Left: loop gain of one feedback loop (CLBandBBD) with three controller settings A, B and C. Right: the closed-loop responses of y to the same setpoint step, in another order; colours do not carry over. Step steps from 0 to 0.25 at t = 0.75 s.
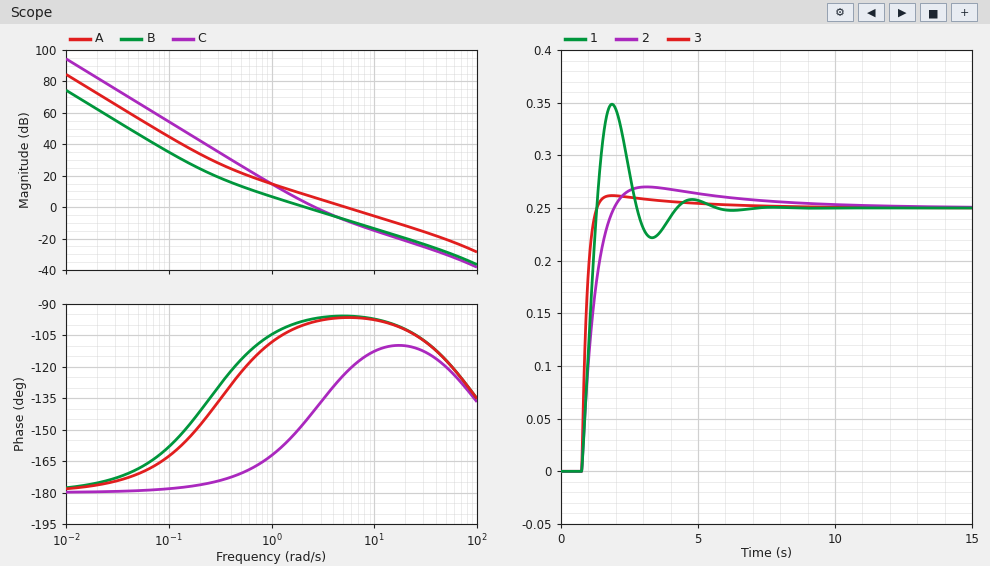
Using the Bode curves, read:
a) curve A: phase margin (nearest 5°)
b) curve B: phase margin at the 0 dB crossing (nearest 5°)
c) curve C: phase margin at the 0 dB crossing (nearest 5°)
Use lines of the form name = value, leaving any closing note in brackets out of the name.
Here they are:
curve A: phase margin = 85°
curve B: phase margin at the 0 dB crossing = 80°
curve C: phase margin at the 0 dB crossing = 40°
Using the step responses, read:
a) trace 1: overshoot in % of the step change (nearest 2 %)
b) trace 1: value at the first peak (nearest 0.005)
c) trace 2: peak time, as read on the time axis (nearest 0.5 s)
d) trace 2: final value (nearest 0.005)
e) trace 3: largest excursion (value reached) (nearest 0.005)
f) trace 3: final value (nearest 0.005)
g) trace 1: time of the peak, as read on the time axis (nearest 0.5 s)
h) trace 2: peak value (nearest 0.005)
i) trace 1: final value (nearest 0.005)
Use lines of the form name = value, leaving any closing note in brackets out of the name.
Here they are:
trace 1: overshoot in % of the step change = 40 %
trace 1: value at the first peak = 0.350
trace 2: peak time, as read on the time axis = 3.0 s
trace 2: final value = 0.250
trace 3: largest excursion (value reached) = 0.260
trace 3: final value = 0.250
trace 1: time of the peak, as read on the time axis = 2.0 s
trace 2: peak value = 0.270
trace 1: final value = 0.250
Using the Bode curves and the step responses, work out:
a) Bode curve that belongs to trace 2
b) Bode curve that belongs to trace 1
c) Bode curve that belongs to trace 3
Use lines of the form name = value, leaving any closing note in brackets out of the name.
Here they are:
Bode curve that belongs to trace 2 = B
Bode curve that belongs to trace 1 = C
Bode curve that belongs to trace 3 = A
